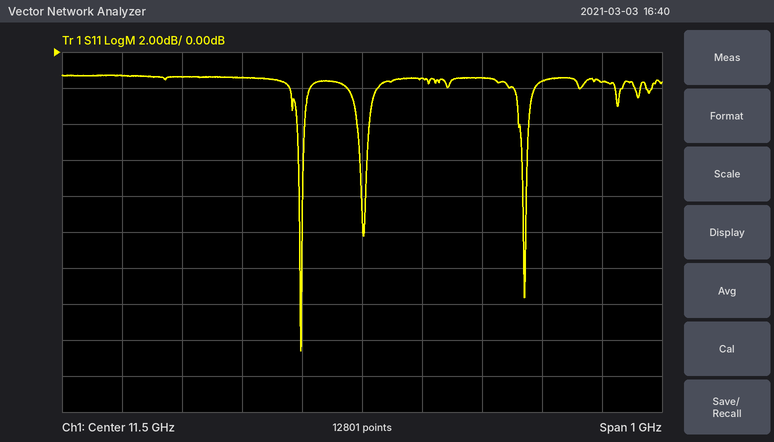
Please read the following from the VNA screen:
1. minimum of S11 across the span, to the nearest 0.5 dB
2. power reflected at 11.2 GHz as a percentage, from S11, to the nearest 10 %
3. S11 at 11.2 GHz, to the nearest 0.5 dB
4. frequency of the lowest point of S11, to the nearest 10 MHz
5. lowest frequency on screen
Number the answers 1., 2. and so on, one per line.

1. -16.5 dB
2. 70 %
3. -1.5 dB
4. 11.40 GHz
5. 11 GHz
